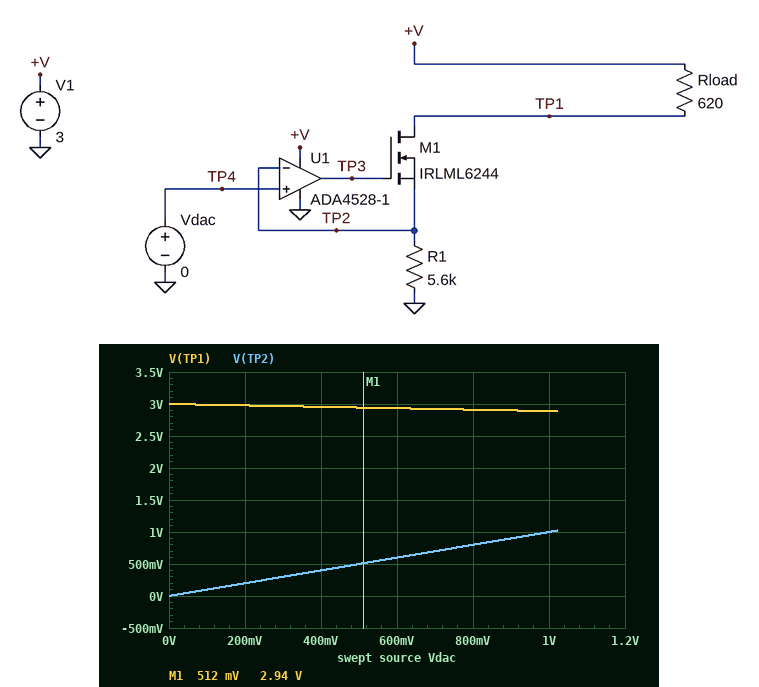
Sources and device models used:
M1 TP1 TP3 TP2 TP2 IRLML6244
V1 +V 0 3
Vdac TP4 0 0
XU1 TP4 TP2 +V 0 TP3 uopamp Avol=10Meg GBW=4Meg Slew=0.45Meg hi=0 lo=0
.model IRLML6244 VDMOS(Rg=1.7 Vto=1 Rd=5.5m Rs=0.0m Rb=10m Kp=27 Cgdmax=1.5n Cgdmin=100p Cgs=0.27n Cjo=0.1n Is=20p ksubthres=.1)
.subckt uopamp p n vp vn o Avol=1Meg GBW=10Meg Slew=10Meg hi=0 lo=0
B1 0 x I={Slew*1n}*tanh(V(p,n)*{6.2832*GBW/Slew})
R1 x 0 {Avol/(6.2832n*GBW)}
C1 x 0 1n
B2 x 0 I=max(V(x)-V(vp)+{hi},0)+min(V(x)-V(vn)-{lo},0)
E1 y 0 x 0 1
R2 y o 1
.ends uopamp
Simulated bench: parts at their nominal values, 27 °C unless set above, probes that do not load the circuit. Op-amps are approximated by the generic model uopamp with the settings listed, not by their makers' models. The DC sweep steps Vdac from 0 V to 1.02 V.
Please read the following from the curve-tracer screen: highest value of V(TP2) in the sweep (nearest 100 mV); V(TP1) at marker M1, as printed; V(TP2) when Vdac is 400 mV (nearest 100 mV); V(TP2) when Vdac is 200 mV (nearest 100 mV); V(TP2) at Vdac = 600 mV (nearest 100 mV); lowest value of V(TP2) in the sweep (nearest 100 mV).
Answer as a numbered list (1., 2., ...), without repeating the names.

1. 1.0 V
2. 2.94 V
3. 400 mV
4. 200 mV
5. 600 mV
6. 0 V
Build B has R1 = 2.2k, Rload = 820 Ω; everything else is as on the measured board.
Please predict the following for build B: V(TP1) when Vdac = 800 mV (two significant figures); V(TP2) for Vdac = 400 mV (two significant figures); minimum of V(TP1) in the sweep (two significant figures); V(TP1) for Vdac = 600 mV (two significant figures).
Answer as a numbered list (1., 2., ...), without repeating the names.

1. 2.7 V
2. 400 mV
3. 2.6 V
4. 2.8 V
